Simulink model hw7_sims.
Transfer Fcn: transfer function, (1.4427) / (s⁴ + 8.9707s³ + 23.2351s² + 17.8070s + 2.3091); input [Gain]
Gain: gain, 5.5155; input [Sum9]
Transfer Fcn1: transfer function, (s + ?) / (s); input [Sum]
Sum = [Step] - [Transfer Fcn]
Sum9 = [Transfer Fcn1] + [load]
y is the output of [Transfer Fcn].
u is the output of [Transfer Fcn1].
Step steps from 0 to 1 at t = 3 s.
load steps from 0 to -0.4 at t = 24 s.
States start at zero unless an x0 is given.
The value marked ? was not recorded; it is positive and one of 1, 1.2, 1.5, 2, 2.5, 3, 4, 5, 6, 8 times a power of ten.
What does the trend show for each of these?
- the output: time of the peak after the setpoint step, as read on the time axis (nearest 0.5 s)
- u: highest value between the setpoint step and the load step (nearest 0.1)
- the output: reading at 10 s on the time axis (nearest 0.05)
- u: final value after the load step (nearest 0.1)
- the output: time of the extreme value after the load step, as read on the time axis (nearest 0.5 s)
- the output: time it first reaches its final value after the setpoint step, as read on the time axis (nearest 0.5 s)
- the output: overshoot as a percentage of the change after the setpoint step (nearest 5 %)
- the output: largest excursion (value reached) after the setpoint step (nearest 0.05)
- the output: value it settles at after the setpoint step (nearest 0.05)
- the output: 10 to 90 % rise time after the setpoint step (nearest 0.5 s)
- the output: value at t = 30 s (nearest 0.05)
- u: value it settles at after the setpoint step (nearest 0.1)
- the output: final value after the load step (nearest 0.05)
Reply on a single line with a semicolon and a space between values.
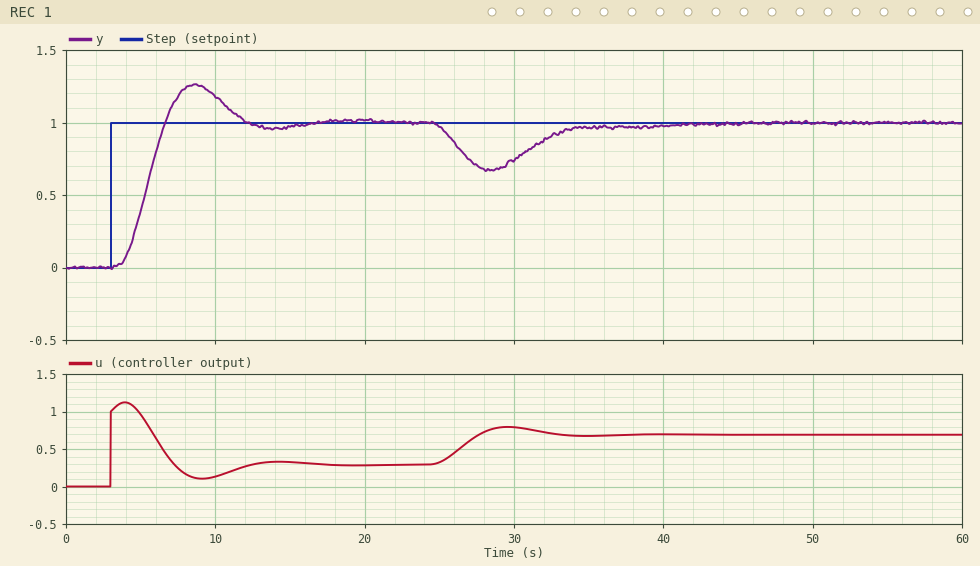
8.5 s; 1.1; 1.20; 0.7; 28.5 s; 6.5 s; 25 %; 1.25; 1.00; 2.0 s; 0.75; 0.3; 1.00
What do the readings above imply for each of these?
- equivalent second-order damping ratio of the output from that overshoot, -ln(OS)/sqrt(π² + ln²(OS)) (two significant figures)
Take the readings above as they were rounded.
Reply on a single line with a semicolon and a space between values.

0.40
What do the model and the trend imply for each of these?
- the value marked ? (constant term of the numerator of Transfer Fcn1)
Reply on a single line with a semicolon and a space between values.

0.2
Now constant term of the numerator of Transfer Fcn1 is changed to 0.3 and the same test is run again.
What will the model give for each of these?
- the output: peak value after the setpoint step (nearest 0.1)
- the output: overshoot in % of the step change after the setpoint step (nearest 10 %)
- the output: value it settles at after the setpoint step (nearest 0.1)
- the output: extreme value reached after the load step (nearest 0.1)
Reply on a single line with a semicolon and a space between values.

1.4; 40 %; 1.0; 0.7
